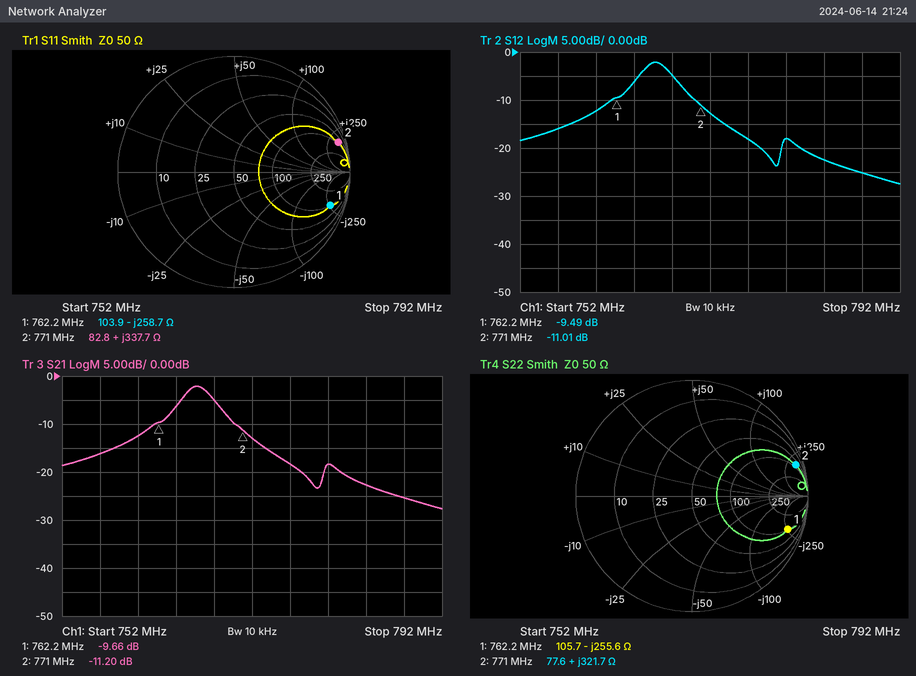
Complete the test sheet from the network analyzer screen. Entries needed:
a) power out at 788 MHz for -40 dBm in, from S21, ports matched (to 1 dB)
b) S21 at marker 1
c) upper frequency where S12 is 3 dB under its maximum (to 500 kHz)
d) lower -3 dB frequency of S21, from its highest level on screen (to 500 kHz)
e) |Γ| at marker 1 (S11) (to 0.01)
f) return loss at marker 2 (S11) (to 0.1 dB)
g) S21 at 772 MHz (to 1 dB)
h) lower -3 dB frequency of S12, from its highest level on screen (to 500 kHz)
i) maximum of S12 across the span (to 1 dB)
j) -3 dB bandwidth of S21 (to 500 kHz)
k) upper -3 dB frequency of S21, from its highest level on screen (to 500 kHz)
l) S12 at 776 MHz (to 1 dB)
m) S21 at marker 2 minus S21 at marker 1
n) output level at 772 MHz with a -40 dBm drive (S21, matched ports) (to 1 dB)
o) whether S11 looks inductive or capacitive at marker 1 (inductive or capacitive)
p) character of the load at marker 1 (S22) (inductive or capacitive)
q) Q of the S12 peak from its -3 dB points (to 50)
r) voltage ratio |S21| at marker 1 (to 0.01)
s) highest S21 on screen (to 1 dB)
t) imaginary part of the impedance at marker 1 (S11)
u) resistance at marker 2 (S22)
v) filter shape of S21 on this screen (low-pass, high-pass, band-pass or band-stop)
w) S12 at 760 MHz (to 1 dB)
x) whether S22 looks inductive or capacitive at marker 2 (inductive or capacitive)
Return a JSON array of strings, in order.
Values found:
["-65 dBm", "-9.66 dB", "768.0 MHz", "764.5 MHz", "0.88", "0.6 dB", "-13 dB", "764.5 MHz", "-2 dB", "3.5 MHz", "768.0 MHz", "-18 dB", "-1.54 dB", "-53 dBm", "capacitive", "capacitive", "200", "0.33", "-2 dB", "-258.7 Ω", "77.6 Ω", "band-pass", "-12 dB", "inductive"]
